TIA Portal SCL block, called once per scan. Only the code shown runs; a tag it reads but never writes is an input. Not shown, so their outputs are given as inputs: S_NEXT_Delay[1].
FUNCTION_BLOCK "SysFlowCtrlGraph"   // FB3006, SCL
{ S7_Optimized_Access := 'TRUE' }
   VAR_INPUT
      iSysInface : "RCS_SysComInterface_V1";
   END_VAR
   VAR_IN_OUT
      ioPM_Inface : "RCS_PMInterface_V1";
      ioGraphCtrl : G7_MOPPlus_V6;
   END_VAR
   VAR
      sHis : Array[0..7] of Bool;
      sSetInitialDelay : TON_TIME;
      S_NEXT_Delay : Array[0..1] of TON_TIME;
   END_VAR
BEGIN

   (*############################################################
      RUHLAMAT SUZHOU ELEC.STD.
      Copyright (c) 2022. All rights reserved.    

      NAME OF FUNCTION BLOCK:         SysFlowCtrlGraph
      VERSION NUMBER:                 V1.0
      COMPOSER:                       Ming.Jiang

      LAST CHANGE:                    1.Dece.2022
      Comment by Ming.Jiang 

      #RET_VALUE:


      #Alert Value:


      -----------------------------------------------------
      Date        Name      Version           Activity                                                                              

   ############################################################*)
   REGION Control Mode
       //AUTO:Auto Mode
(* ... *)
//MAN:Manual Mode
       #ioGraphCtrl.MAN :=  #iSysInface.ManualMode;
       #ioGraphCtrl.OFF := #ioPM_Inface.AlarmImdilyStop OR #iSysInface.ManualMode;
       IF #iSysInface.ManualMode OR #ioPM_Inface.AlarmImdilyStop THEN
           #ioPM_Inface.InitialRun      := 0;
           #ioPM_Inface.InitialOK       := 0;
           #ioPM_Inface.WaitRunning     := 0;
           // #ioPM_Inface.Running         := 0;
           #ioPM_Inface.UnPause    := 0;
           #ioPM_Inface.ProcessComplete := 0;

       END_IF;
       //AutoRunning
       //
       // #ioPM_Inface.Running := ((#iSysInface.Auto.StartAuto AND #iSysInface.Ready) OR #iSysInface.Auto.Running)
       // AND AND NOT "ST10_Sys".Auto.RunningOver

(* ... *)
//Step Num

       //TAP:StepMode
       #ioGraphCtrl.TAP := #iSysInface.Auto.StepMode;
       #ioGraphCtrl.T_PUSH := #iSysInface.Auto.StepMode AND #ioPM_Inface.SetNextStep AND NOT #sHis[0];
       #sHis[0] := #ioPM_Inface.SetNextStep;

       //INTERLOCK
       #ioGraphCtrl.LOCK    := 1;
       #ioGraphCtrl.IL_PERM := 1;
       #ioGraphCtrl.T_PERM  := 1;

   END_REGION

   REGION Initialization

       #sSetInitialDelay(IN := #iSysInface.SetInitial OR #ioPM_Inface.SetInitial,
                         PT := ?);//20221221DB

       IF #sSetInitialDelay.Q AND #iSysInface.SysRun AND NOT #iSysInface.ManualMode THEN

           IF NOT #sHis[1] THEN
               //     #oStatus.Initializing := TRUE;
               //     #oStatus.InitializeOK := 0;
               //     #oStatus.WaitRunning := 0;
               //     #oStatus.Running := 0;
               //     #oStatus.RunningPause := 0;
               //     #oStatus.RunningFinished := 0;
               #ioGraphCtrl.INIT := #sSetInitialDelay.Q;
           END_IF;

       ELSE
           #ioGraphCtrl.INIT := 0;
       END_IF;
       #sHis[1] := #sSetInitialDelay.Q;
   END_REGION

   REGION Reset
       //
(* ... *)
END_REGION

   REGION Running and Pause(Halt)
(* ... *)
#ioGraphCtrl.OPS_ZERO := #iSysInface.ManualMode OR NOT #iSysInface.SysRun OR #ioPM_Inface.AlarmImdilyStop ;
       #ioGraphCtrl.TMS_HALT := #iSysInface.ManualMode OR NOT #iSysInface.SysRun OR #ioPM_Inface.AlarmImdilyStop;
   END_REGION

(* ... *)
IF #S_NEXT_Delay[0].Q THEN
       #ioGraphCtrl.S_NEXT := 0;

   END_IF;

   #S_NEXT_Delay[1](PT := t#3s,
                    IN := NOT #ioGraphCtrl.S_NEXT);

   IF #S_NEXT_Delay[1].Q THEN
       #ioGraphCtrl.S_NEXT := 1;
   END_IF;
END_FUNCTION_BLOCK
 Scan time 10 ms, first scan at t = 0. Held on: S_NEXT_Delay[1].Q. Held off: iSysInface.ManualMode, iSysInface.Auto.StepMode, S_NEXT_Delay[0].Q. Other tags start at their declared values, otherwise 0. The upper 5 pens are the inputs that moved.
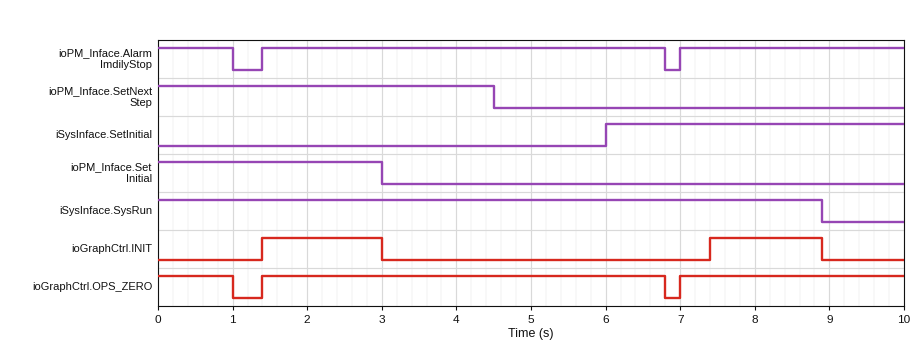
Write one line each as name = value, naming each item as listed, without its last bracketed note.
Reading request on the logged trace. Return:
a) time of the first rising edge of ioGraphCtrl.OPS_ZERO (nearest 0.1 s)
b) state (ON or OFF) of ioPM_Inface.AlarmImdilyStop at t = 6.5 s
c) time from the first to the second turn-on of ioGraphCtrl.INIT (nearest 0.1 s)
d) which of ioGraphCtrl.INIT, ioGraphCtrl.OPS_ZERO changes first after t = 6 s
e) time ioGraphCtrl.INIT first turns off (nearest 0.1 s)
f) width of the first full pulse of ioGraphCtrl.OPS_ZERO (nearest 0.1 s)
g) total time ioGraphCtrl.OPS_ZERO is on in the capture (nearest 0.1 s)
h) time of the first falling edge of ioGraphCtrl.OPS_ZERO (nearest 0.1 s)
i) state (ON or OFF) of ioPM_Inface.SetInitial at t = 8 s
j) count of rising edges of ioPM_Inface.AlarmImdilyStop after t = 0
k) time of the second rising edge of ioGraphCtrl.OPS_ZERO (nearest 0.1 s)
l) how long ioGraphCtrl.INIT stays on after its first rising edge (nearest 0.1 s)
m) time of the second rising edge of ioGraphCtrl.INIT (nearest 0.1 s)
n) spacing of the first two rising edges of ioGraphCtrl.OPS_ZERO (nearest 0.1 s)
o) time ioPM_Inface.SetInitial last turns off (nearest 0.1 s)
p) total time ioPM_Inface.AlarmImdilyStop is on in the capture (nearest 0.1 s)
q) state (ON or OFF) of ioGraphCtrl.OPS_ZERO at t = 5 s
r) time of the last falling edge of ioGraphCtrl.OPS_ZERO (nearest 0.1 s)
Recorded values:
time of the first rising edge of ioGraphCtrl.OPS_ZERO = 1.4 s
state (ON or OFF) of ioPM_Inface.AlarmImdilyStop at t = 6.5 s = ON
time from the first to the second turn-on of ioGraphCtrl.INIT = 6.0 s
which of ioGraphCtrl.INIT, ioGraphCtrl.OPS_ZERO changes first after t = 6 s = ioGraphCtrl.OPS_ZERO
time ioGraphCtrl.INIT first turns off = 3.0 s
width of the first full pulse of ioGraphCtrl.OPS_ZERO = 5.4 s
total time ioGraphCtrl.OPS_ZERO is on in the capture = 9.4 s
time of the first falling edge of ioGraphCtrl.OPS_ZERO = 1.0 s
state (ON or OFF) of ioPM_Inface.SetInitial at t = 8 s = OFF
count of rising edges of ioPM_Inface.AlarmImdilyStop after t = 0 = 2
time of the second rising edge of ioGraphCtrl.OPS_ZERO = 7.0 s
how long ioGraphCtrl.INIT stays on after its first rising edge = 1.6 s
time of the second rising edge of ioGraphCtrl.INIT = 7.4 s
spacing of the first two rising edges of ioGraphCtrl.OPS_ZERO = 5.6 s
time ioPM_Inface.SetInitial last turns off = 3.0 s
total time ioPM_Inface.AlarmImdilyStop is on in the capture = 9.4 s
state (ON or OFF) of ioGraphCtrl.OPS_ZERO at t = 5 s = ON
time of the last falling edge of ioGraphCtrl.OPS_ZERO = 6.8 s
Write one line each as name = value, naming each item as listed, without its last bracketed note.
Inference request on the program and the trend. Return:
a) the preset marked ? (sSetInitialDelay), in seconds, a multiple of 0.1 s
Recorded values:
the preset marked ? (sSetInitialDelay), in seconds, a multiple of 0.1 s = 1.4 s
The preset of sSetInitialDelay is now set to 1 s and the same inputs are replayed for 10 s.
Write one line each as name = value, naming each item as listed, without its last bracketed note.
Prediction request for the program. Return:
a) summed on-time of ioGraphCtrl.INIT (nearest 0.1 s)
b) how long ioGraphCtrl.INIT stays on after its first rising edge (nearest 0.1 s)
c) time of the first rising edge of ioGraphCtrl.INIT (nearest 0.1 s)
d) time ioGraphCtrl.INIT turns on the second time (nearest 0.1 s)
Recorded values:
summed on-time of ioGraphCtrl.INIT = 3.9 s
how long ioGraphCtrl.INIT stays on after its first rising edge = 2.0 s
time of the first rising edge of ioGraphCtrl.INIT = 1.0 s
time ioGraphCtrl.INIT turns on the second time = 7.0 s
